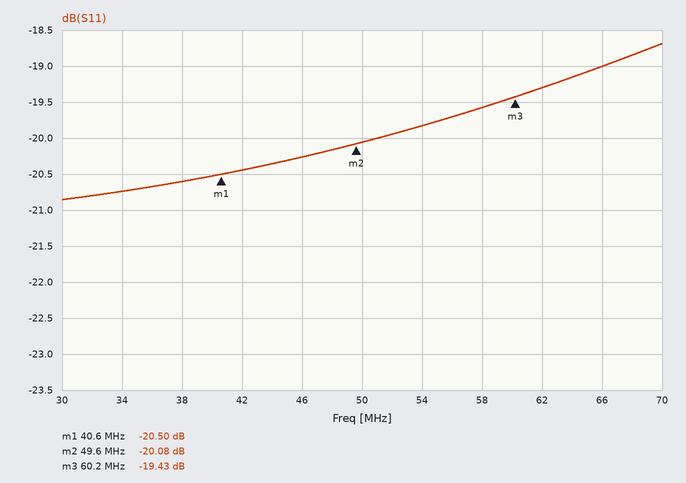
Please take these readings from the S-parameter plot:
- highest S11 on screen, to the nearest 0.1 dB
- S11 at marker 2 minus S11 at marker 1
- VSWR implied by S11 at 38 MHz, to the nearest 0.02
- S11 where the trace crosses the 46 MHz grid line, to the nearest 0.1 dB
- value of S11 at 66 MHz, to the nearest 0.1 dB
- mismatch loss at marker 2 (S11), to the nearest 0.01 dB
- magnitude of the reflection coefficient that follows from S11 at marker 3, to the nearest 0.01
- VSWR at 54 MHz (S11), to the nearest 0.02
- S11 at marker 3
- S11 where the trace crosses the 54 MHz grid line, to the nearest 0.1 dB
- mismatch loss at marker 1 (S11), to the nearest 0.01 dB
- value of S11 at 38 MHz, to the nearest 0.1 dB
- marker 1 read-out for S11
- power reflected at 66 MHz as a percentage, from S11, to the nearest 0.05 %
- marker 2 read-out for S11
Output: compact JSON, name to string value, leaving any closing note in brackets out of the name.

{"highest S11 on screen, to the nearest 0.1 dB": "-18.7 dB", "S11 at marker 2 minus S11 at marker 1": "0.42 dB", "VSWR implied by S11 at 38 MHz, to the nearest 0.02": "1.20", "S11 where the trace crosses the 46 MHz grid line, to the nearest 0.1 dB": "-20.3 dB", "value of S11 at 66 MHz, to the nearest 0.1 dB": "-19.0 dB", "mismatch loss at marker 2 (S11), to the nearest 0.01 dB": "0.04 dB", "magnitude of the reflection coefficient that follows from S11 at marker 3, to the nearest 0.01": "0.11", "VSWR at 54 MHz (S11), to the nearest 0.02": "1.22", "S11 at marker 3": "-19.43 dB", "S11 where the trace crosses the 54 MHz grid line, to the nearest 0.1 dB": "-19.8 dB", "mismatch loss at marker 1 (S11), to the nearest 0.01 dB": "0.04 dB", "value of S11 at 38 MHz, to the nearest 0.1 dB": "-20.6 dB", "marker 1 read-out for S11": "-20.50 dB", "power reflected at 66 MHz as a percentage, from S11, to the nearest 0.05 %": "1.25 %", "marker 2 read-out for S11": "-20.08 dB"}
